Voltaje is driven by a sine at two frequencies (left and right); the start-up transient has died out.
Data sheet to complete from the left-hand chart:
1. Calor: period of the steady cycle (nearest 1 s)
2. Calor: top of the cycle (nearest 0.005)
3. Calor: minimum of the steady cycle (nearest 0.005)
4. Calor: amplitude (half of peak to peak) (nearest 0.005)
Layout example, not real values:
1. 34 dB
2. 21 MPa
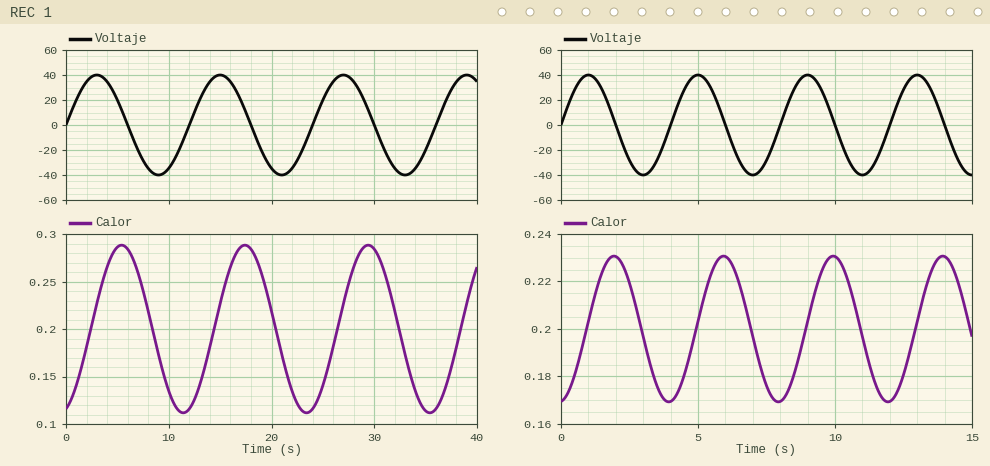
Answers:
1. 12 s
2. 0.290
3. 0.110
4. 0.090
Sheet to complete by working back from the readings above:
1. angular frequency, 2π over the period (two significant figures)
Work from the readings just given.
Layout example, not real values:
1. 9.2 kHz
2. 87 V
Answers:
1. 0.52 rad/s
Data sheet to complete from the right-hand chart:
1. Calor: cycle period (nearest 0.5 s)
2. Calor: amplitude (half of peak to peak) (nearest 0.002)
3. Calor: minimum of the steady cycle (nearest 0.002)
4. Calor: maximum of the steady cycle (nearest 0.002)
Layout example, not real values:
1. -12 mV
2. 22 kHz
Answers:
1. 4.0 s
2. 0.030
3. 0.170
4. 0.230
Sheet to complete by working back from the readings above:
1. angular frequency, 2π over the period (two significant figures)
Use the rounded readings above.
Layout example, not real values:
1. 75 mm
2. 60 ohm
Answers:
1. 1.6 rad/s
